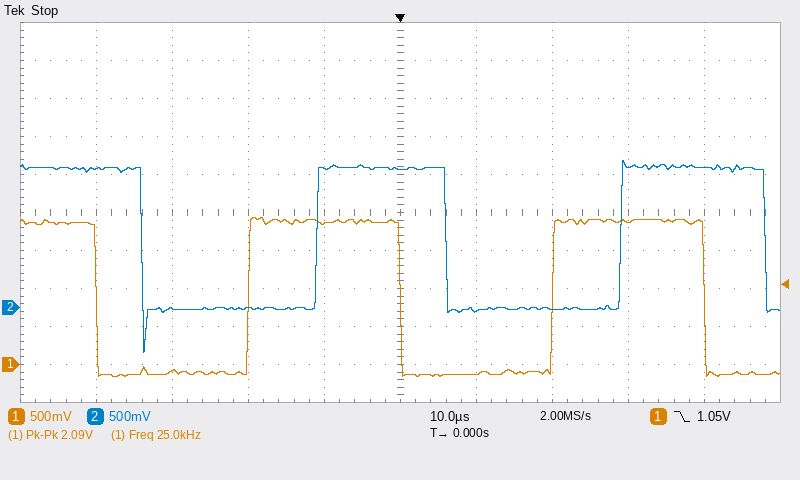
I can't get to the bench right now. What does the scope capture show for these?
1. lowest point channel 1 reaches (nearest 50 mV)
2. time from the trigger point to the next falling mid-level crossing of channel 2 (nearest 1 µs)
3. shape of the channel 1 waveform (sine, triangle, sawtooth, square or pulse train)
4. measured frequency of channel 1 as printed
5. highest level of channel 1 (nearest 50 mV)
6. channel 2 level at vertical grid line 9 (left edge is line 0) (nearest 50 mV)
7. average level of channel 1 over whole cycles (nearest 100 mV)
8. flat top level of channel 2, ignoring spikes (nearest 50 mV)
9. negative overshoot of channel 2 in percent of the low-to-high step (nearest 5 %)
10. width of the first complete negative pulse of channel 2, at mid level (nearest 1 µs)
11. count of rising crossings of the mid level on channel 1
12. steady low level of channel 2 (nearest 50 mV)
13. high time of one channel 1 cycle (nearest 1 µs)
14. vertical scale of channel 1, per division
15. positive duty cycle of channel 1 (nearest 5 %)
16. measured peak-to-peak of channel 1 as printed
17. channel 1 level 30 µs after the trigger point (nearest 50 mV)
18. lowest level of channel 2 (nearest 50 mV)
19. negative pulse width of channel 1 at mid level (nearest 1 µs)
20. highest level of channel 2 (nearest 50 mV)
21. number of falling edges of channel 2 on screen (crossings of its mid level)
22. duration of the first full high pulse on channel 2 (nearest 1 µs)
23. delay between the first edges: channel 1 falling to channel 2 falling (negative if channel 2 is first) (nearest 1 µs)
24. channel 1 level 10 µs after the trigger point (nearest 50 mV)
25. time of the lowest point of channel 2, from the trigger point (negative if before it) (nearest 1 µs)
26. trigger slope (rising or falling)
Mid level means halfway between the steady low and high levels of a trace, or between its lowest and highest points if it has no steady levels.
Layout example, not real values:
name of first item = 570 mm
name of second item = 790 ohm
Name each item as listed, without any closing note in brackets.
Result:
lowest point channel 1 reaches = -150 mV
time from the trigger point to the next falling mid-level crossing of channel 2 = 6 µs
shape of the channel 1 waveform = square
measured frequency of channel 1 as printed = 25.0 kHz
highest level of channel 1 = 1.95 V
channel 2 level at vertical grid line 9 (left edge is line 0) = 1.85 V
average level of channel 1 over whole cycles = 900 mV
flat top level of channel 2, ignoring spikes = 1.85 V
negative overshoot of channel 2 in percent of the low-to-high step = 30 %
width of the first complete negative pulse of channel 2, at mid level = 23 µs
count of rising crossings of the mid level on channel 1 = 2
steady low level of channel 2 = -50 mV
high time of one channel 1 cycle = 20 µs
vertical scale of channel 1, per division = 500 mV
positive duty cycle of channel 1 = 50 %
measured peak-to-peak of channel 1 as printed = 2.09 V
channel 1 level 30 µs after the trigger point = 1.90 V
lowest level of channel 2 = -600 mV
negative pulse width of channel 1 at mid level = 20 µs
highest level of channel 2 = 1.95 V
number of falling edges of channel 2 on screen = 3
duration of the first full high pulse on channel 2 = 17 µs
delay between the first edges: channel 1 falling to channel 2 falling (negative if channel 2 is first) = +6 µs
channel 1 level 10 µs after the trigger point = -100 mV
time of the lowest point of channel 2, from the trigger point (negative if before it) = -34 µs
trigger slope = falling
